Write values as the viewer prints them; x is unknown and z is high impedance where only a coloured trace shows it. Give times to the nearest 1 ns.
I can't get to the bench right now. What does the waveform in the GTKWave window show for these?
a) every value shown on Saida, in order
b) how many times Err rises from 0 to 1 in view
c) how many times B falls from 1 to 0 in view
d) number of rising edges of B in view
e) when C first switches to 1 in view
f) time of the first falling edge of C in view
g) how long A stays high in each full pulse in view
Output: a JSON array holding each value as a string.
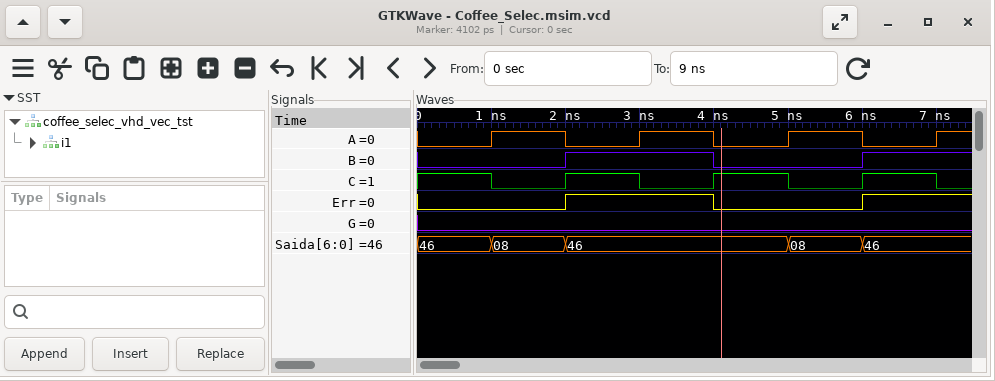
["46, 08, 46, 08, 46", "2", "1", "2", "2 ns", "1 ns", "1 ns, 1 ns, 1 ns"]
